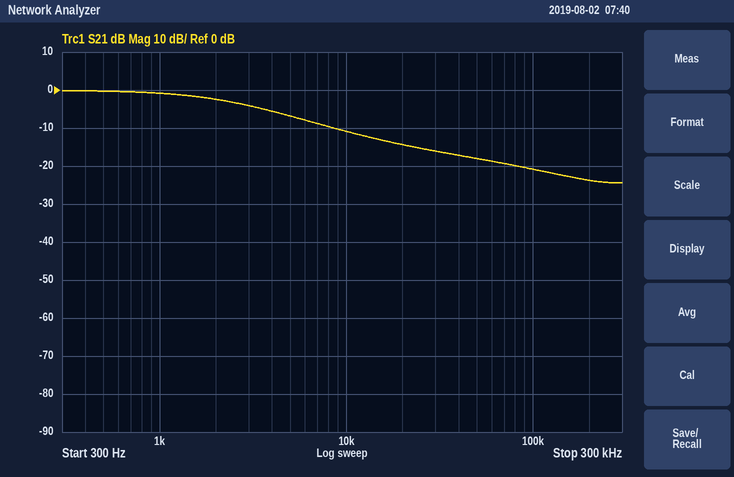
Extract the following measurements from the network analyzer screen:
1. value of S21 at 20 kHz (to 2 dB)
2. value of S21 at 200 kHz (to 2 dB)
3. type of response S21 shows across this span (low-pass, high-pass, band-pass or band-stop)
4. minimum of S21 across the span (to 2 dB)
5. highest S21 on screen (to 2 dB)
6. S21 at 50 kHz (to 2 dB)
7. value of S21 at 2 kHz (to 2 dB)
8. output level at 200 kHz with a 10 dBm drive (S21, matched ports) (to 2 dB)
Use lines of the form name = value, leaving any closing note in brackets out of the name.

value of S21 at 20 kHz = -14 dB
value of S21 at 200 kHz = -24 dB
type of response S21 shows across this span = low-pass
minimum of S21 across the span = -24 dB
highest S21 on screen = 0 dB
S21 at 50 kHz = -18 dB
value of S21 at 2 kHz = -2 dB
output level at 200 kHz with a 10 dBm drive (S21, matched ports) = -14 dBm
